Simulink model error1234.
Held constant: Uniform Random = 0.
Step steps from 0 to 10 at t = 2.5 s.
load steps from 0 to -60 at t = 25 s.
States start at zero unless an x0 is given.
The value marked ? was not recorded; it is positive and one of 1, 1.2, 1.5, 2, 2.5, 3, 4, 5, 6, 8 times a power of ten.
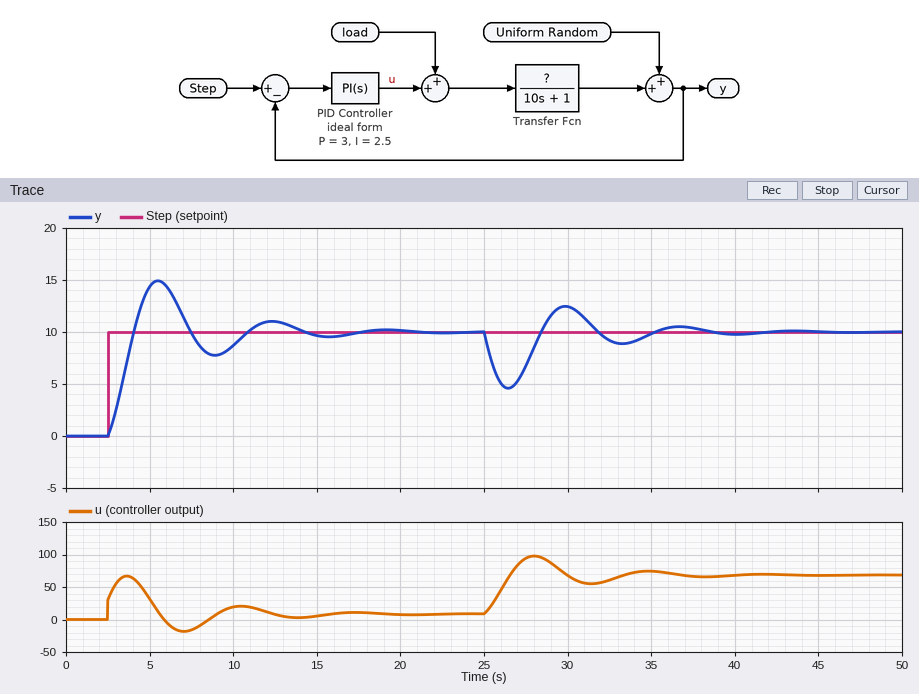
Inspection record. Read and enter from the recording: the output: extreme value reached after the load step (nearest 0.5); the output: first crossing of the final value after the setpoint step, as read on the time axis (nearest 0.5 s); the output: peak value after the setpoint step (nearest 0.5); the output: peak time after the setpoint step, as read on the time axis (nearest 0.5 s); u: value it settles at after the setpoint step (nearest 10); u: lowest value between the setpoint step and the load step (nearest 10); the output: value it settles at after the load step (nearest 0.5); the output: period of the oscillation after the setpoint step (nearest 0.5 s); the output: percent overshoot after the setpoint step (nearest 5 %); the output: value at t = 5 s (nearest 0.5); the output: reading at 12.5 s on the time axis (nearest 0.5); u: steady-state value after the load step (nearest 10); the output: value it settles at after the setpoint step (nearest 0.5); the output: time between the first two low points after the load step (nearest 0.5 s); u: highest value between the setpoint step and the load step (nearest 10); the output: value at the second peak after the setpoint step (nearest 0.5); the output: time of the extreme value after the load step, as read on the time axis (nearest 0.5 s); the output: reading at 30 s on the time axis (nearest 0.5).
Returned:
4.5
4.0 s
15.0
5.5 s
10
-20
10.0
7.0 s
50 %
14.5
11.0
70
10.0
7.0 s
70
11.0
26.5 s
12.5
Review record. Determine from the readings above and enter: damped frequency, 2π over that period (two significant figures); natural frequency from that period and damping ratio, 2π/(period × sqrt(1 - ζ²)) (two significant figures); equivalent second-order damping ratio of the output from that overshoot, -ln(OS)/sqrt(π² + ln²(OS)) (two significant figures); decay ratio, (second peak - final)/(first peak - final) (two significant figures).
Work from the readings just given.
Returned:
0.90 rad/s
0.92 rad/s
0.22
0.20
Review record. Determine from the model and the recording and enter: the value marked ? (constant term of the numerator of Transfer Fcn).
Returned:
1.2
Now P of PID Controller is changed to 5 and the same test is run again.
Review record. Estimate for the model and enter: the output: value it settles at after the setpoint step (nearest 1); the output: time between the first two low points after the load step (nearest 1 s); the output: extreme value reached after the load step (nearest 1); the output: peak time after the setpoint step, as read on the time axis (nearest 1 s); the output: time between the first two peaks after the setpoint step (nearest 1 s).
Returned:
10
5 s
6
5 s
5 s
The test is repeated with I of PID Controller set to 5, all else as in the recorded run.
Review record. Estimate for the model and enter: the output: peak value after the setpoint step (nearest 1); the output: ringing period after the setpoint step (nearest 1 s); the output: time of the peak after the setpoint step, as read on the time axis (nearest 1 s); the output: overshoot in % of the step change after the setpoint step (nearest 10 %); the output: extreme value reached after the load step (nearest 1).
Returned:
16
5 s
5 s
60 %
6
